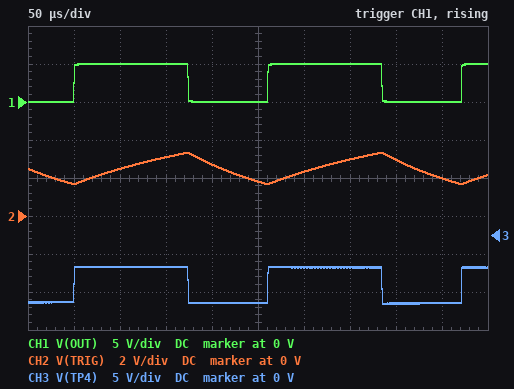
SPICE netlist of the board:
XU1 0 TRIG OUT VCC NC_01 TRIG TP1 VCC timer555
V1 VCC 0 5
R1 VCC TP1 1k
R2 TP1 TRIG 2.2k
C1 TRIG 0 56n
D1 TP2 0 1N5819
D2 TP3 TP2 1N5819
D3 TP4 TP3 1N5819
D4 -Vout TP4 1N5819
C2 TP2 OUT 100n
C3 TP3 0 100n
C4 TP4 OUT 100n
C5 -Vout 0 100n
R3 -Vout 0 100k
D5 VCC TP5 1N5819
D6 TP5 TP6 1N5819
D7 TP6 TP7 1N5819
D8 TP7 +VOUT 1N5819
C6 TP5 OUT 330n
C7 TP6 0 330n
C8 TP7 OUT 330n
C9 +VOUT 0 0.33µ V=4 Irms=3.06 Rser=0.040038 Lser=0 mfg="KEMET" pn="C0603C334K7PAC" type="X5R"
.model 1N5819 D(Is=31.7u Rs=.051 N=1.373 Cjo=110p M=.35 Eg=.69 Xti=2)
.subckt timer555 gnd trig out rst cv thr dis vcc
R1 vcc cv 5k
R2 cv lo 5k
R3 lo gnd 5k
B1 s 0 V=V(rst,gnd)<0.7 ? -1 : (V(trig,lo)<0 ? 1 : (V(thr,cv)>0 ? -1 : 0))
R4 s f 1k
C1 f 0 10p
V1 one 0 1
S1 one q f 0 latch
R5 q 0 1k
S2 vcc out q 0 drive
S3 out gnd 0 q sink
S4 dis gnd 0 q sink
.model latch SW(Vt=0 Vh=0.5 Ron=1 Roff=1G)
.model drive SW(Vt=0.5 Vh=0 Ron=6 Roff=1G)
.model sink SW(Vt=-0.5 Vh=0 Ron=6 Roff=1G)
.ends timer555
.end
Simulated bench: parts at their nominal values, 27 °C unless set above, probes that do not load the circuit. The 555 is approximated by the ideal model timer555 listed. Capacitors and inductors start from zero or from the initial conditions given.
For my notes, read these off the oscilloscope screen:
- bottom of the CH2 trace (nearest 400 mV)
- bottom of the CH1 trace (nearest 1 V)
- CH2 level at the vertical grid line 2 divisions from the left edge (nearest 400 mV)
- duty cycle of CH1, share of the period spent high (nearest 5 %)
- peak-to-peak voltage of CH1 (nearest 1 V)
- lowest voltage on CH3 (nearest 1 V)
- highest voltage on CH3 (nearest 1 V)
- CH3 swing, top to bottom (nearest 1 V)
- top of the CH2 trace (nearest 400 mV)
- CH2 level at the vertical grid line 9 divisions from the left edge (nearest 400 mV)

1.6 V
0 V
2.4 V
60 %
5 V
-9 V
-4 V
5 V
3.2 V
2.0 V
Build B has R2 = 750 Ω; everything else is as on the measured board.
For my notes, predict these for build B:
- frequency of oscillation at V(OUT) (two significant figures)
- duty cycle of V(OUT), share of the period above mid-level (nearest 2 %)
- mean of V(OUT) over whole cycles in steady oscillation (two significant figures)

10 kHz
70 %
3.5 V
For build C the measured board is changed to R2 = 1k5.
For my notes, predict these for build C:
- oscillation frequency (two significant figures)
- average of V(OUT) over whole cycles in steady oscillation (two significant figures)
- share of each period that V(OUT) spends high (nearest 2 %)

6.4 kHz
3.1 V
62 %
